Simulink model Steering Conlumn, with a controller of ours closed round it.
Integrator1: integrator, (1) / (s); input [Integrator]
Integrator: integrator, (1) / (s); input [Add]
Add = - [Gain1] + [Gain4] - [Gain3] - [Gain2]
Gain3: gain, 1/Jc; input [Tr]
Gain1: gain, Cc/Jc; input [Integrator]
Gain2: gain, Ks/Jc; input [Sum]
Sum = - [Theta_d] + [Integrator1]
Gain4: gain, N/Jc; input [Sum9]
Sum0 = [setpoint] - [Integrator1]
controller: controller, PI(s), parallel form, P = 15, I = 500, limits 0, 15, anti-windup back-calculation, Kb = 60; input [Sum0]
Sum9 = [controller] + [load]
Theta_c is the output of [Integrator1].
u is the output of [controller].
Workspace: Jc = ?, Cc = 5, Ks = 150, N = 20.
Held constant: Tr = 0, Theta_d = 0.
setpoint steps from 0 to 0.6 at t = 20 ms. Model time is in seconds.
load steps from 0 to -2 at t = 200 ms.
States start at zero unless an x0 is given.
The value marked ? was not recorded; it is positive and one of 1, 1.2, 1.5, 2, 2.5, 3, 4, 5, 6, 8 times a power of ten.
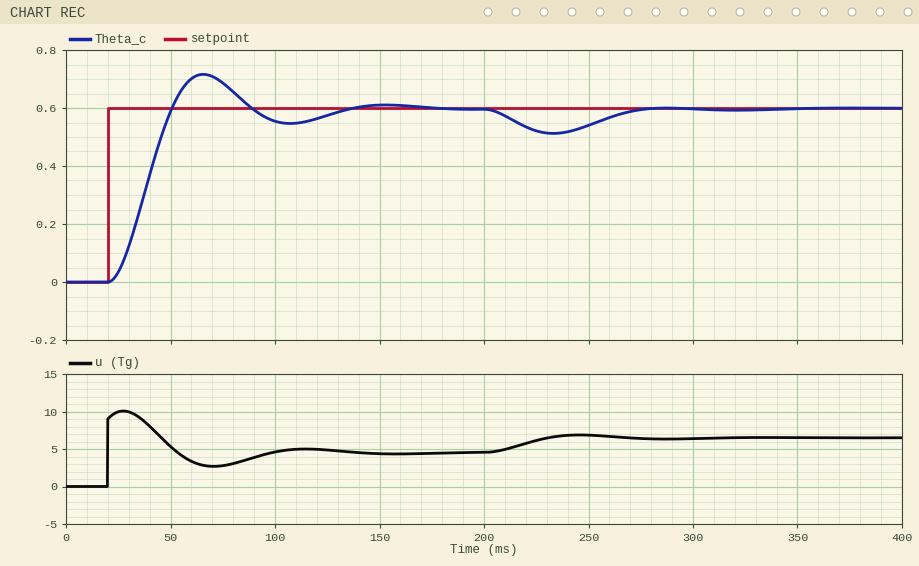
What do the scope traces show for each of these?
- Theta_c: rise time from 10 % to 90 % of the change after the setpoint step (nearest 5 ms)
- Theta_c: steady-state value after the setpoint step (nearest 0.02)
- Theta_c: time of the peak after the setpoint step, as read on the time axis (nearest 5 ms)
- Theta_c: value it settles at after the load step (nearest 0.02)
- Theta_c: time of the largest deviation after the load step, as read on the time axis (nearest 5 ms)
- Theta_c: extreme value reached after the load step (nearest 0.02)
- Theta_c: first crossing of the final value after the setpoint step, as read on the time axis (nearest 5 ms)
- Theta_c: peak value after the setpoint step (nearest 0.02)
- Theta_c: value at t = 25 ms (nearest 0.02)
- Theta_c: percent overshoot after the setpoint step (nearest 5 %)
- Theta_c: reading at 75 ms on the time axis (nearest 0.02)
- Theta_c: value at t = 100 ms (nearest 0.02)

20 ms
0.60
65 ms
0.60
235 ms
0.52
50 ms
0.72
0.04
20 %
0.68
0.56
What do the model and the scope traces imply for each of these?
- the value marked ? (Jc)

0.06
